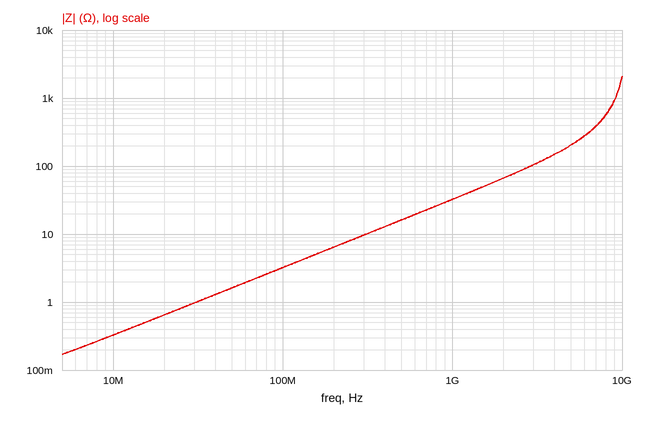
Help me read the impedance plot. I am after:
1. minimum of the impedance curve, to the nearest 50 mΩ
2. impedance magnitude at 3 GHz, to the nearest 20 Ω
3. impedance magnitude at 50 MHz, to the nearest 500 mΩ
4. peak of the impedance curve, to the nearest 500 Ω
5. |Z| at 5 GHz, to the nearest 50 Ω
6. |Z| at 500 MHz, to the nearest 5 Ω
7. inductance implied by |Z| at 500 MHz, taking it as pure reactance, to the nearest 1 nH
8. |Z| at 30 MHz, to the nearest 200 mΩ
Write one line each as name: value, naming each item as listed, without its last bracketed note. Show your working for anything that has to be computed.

minimum of the impedance curve, to the nearest 50 mΩ: 150 mΩ
impedance magnitude at 3 GHz, to the nearest 20 Ω: 100 Ω
impedance magnitude at 50 MHz, to the nearest 500 mΩ: 1.5 Ω
peak of the impedance curve, to the nearest 500 Ω: 2.0 kΩ
|Z| at 5 GHz, to the nearest 50 Ω: 200 Ω
|Z| at 500 MHz, to the nearest 5 Ω: 15 Ω
inductance implied by |Z| at 500 MHz, taking it as pure reactance, to the nearest 1 nH: L = 15 Ω/(2π × 500 MHz) ≈ 5 nH
|Z| at 30 MHz, to the nearest 200 mΩ: 1.0 Ω
